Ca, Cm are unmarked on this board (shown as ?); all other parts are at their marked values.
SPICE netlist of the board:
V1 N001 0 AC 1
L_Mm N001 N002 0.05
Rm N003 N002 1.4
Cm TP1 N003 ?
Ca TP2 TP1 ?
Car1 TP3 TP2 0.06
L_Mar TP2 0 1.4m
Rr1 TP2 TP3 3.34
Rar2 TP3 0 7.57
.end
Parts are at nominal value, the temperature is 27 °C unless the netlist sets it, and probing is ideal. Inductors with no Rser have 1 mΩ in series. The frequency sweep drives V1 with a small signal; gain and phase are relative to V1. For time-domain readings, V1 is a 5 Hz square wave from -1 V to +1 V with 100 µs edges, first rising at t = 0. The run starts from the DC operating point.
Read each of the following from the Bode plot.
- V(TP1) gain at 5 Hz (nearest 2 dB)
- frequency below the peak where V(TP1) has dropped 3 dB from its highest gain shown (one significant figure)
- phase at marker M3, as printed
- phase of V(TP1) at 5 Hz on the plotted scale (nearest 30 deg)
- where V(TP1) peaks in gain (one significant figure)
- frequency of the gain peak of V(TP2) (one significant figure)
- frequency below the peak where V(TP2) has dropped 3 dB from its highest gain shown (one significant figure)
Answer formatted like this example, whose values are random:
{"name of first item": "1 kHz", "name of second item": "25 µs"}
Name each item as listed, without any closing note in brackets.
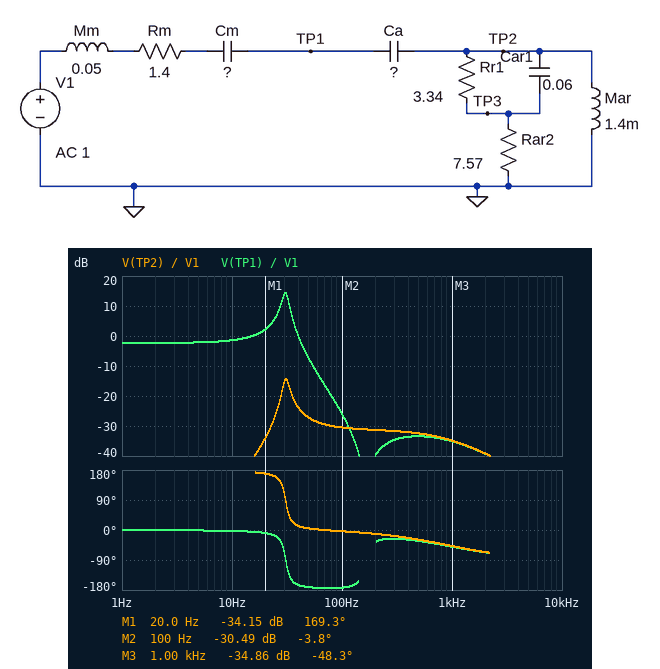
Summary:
{"V(TP1) gain at 5 Hz": "-2 dB", "frequency below the peak where V(TP1) has dropped 3 dB from its highest gain shown": "30 Hz", "phase at marker M3, as printed": "-48.3 deg", "phase of V(TP1) at 5 Hz on the plotted scale": "0 deg", "where V(TP1) peaks in gain": "30 Hz", "frequency of the gain peak of V(TP2)": "30 Hz", "frequency below the peak where V(TP2) has dropped 3 dB from its highest gain shown": "30 Hz"}
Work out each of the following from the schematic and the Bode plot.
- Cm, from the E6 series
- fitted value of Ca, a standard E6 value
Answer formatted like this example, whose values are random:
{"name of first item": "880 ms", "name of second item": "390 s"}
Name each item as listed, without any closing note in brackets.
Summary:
{"Cm, from the E6 series": "2.2 mF", "fitted value of Ca, a standard E6 value": "680 µF"}
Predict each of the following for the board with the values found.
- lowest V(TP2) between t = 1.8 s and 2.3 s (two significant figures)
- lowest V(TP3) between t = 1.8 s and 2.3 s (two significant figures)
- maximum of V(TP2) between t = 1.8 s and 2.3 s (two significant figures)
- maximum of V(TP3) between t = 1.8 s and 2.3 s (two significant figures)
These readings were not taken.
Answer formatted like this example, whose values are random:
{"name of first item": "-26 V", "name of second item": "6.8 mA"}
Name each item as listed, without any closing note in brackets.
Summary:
{"lowest V(TP2) between t = 1.8 s and 2.3 s": "-43 mV", "lowest V(TP3) between t = 1.8 s and 2.3 s": "-43 mV", "maximum of V(TP2) between t = 1.8 s and 2.3 s": "43 mV", "maximum of V(TP3) between t = 1.8 s and 2.3 s": "43 mV"}
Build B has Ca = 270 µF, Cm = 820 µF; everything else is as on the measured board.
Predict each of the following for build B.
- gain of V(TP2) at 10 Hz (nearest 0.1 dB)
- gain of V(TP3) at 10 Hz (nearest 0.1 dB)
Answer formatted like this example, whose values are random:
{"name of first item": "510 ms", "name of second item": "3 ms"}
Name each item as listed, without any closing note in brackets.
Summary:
{"gain of V(TP2) at 10 Hz": "-58.6 dB", "gain of V(TP3) at 10 Hz": "-58.7 dB"}
